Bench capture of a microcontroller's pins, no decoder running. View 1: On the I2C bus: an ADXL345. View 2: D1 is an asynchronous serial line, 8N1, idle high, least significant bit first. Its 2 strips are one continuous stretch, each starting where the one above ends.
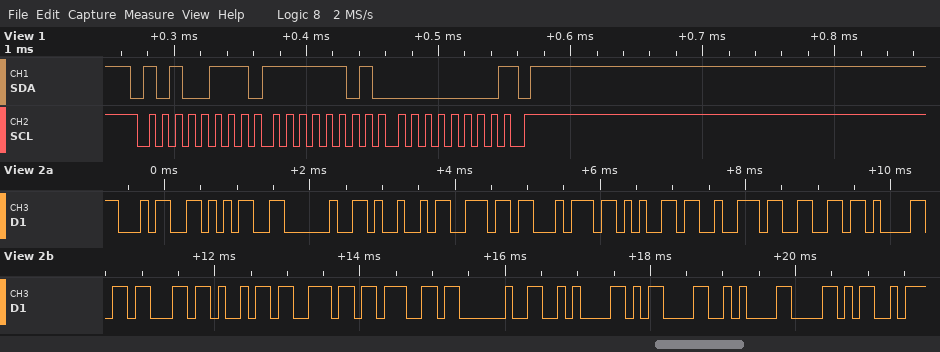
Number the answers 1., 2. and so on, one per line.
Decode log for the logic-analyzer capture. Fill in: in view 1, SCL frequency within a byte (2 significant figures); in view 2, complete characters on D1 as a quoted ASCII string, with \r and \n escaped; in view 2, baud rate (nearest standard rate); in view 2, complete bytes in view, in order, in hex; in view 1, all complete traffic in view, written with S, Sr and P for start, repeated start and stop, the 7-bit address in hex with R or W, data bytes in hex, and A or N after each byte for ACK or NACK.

1. 100 kHz
2. "45 Interfacing \n\r\nX"
3. 9600 baud
4. 34 35 20 49 6E 74 65 72 66 61 63 69 6E 67 20 0A 0D 0A 58
5. S 53R A FD A 00 N P
